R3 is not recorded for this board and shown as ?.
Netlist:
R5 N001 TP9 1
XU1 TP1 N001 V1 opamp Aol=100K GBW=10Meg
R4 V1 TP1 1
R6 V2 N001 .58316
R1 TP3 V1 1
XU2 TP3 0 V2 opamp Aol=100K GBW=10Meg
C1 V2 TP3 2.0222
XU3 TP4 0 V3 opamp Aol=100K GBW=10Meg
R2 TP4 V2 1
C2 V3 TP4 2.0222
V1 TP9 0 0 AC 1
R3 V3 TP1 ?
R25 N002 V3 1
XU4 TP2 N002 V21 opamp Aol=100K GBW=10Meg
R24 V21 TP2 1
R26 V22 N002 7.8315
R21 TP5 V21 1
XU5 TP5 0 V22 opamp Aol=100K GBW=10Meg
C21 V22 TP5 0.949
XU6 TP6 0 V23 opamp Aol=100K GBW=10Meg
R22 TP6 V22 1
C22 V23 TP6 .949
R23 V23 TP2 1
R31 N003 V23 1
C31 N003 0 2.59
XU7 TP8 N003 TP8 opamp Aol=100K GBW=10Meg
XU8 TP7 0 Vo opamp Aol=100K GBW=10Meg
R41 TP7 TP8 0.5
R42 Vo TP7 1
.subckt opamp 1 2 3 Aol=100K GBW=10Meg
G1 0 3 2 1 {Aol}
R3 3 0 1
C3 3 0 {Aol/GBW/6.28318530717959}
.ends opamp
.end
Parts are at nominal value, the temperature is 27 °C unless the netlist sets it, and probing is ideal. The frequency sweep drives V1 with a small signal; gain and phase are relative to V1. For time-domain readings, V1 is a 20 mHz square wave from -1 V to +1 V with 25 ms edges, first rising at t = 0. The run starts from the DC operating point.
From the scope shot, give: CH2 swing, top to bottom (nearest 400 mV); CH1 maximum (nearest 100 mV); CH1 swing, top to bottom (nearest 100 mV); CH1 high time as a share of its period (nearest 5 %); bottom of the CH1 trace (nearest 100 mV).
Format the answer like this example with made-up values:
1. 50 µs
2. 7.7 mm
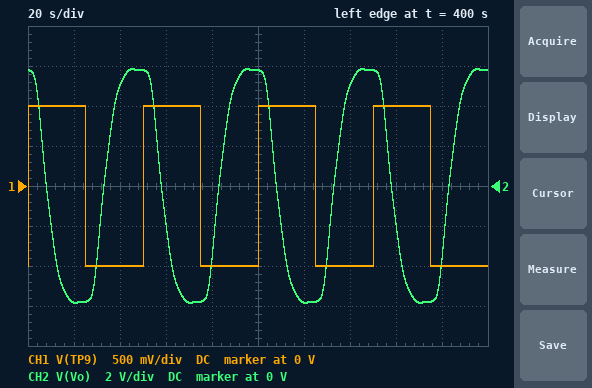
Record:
1. 11.6 V
2. 1.0 V
3. 2.0 V
4. 50 %
5. -1.0 V
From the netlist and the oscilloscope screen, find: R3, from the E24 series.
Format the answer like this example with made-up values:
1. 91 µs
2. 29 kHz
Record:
1. 3.3 Ω
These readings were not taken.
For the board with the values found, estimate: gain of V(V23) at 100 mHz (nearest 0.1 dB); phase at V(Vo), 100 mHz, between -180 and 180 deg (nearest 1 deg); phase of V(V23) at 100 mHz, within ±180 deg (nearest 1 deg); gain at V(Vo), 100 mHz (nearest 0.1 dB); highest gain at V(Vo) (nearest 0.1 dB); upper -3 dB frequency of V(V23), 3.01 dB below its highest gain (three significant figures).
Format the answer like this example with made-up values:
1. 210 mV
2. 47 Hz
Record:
1. -2.3 dB
2. -32 deg
3. -153 deg
4. -1.9 dB
5. 15.0 dB
6. 43.9 mHz
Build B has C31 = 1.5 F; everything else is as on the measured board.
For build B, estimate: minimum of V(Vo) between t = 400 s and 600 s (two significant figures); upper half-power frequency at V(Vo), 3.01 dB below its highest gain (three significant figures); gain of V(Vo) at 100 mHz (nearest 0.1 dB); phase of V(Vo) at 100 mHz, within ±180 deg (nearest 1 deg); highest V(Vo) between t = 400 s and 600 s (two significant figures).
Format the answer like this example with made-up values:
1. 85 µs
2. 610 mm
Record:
1. -6.0 V
2. 40.4 mHz
3. 1.0 dB
4. -17 deg
5. 6.0 V
